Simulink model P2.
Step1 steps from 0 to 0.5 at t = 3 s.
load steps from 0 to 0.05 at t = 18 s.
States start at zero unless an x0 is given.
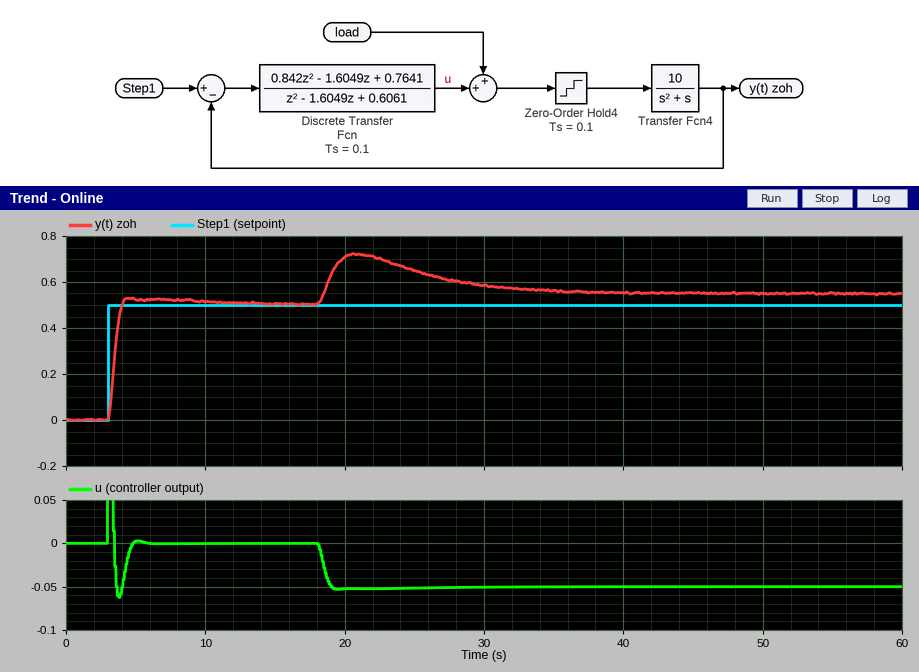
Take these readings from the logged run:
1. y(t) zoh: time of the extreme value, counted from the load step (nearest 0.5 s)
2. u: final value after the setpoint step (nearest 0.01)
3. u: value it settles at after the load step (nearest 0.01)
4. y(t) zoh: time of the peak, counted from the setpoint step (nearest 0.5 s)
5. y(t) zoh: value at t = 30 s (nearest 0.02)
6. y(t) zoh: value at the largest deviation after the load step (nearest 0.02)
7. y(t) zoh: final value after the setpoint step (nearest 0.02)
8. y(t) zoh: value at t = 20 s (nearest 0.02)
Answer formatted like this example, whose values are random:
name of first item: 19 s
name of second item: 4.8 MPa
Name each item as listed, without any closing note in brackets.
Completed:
y(t) zoh: time of the extreme value, counted from the load step: 3.0 s
u: final value after the setpoint step: 0.00
u: value it settles at after the load step: -0.05
y(t) zoh: time of the peak, counted from the setpoint step: 1.5 s
y(t) zoh: value at t = 30 s: 0.58
y(t) zoh: value at the largest deviation after the load step: 0.72
y(t) zoh: final value after the setpoint step: 0.50
y(t) zoh: value at t = 20 s: 0.70
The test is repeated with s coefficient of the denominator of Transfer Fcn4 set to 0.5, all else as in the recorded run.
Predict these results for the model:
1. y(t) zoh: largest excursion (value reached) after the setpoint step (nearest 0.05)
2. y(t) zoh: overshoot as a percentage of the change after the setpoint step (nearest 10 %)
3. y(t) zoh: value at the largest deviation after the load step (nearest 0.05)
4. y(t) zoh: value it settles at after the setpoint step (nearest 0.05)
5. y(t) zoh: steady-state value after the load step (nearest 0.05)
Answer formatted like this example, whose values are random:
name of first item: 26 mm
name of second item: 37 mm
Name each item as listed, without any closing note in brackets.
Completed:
y(t) zoh: largest excursion (value reached) after the setpoint step: 0.60
y(t) zoh: overshoot as a percentage of the change after the setpoint step: 20 %
y(t) zoh: value at the largest deviation after the load step: 0.75
y(t) zoh: value it settles at after the setpoint step: 0.50
y(t) zoh: steady-state value after the load step: 0.55
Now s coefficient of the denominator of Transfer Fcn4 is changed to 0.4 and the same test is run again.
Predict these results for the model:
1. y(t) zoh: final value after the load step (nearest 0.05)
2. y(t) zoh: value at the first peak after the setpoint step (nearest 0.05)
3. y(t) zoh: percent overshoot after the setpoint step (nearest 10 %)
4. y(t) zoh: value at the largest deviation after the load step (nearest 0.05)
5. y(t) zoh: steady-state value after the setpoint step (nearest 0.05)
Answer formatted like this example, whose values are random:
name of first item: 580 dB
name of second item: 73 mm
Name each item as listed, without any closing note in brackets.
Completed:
y(t) zoh: final value after the load step: 0.55
y(t) zoh: value at the first peak after the setpoint step: 0.65
y(t) zoh: percent overshoot after the setpoint step: 30 %
y(t) zoh: value at the largest deviation after the load step: 0.75
y(t) zoh: steady-state value after the setpoint step: 0.50
